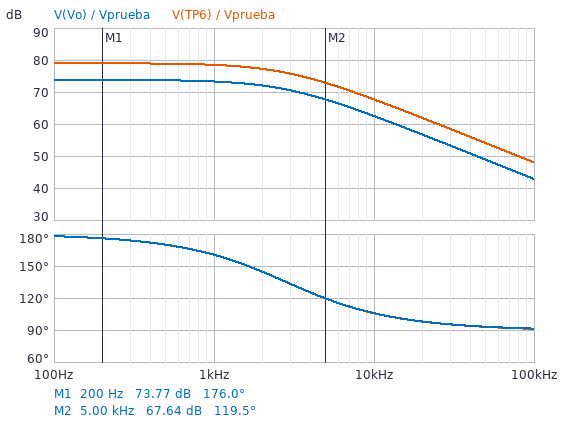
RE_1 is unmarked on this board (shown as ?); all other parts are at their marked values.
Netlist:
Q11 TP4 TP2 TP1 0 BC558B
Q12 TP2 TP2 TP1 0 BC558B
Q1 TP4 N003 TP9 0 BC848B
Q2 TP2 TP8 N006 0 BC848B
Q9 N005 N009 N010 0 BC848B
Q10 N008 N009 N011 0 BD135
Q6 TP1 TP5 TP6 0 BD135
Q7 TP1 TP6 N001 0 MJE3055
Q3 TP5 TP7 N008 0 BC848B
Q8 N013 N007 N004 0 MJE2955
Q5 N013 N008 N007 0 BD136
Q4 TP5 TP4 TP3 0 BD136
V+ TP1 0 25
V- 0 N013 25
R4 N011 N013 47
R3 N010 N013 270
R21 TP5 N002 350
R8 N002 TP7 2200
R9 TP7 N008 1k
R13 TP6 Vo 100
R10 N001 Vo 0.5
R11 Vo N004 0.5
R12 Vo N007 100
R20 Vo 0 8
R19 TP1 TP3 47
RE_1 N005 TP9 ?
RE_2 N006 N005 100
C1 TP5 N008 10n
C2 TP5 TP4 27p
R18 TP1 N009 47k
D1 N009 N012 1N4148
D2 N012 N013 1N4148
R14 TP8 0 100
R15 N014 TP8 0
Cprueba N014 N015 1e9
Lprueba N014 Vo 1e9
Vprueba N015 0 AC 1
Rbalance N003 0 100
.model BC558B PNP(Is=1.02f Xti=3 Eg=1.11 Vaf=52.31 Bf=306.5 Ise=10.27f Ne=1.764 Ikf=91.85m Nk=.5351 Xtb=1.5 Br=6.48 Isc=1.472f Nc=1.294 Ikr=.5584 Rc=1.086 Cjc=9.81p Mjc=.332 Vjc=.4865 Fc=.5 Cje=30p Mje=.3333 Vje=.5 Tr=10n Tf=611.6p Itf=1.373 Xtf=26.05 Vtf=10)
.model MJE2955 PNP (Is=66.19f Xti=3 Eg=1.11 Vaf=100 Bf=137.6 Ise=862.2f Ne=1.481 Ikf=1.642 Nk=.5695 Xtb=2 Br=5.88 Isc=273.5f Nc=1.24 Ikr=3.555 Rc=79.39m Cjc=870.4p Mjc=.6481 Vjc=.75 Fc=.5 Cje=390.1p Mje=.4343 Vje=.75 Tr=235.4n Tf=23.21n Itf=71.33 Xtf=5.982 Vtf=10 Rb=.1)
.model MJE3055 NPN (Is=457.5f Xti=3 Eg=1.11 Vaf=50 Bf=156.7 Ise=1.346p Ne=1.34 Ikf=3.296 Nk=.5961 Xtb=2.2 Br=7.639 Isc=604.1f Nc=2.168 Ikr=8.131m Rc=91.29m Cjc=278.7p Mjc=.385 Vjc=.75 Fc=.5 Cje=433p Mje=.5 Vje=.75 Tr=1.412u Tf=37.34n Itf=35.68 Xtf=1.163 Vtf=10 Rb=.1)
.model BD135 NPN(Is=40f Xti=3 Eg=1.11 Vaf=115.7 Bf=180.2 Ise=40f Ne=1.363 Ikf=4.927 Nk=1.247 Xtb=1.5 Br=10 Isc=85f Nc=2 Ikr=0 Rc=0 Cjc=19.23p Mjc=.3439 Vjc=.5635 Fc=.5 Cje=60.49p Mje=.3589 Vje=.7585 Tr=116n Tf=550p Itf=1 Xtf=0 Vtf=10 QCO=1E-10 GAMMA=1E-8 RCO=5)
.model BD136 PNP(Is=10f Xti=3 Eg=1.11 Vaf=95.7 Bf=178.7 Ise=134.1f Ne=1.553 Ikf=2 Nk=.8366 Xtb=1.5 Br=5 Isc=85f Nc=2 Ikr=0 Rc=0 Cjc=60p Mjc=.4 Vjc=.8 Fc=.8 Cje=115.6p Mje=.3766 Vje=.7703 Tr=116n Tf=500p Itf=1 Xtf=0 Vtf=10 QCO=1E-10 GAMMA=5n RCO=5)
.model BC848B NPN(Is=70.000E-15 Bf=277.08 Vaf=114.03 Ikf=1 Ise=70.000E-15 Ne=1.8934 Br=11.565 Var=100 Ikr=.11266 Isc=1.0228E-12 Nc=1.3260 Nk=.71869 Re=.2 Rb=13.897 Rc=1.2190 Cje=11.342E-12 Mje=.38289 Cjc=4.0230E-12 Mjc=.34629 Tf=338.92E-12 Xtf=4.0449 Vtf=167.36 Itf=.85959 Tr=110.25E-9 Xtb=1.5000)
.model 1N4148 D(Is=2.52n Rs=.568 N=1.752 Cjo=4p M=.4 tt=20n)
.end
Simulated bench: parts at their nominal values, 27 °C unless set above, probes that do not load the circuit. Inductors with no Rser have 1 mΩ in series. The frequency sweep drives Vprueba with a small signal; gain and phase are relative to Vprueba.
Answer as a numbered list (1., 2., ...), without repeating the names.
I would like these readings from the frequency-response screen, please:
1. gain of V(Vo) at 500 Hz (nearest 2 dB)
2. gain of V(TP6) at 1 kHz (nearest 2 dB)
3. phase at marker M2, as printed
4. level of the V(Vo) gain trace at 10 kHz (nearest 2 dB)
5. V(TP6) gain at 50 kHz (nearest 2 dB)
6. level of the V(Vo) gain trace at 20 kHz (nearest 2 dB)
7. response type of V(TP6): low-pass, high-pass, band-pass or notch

1. 74 dB
2. 78 dB
3. 119.5 deg
4. 62 dB
5. 54 dB
6. 56 dB
7. low-pass
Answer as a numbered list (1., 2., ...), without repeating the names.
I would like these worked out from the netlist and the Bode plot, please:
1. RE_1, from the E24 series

1. 130 Ω
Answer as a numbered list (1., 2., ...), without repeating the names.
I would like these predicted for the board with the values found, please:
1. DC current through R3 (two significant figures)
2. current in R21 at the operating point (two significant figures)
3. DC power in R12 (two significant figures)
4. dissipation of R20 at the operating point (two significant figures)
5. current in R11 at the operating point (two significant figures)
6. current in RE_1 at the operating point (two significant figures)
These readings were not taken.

1. 2.0 mA
2. 700 µA
3. 4.0 mW
4. 190 µW
5. 3.6 mA
6. 1.0 mA
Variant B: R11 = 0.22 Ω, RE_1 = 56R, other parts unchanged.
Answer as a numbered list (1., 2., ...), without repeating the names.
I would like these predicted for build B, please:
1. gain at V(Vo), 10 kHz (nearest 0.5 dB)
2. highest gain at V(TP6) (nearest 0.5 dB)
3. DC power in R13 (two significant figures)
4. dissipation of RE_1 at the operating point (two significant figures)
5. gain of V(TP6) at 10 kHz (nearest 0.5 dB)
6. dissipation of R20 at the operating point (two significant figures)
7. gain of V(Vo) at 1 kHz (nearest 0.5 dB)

1. 66.0 dB
2. 82.5 dB
3. 3.4 mW
4. 61 µW
5. 70.5 dB
6. 180 µW
7. 77.0 dB
